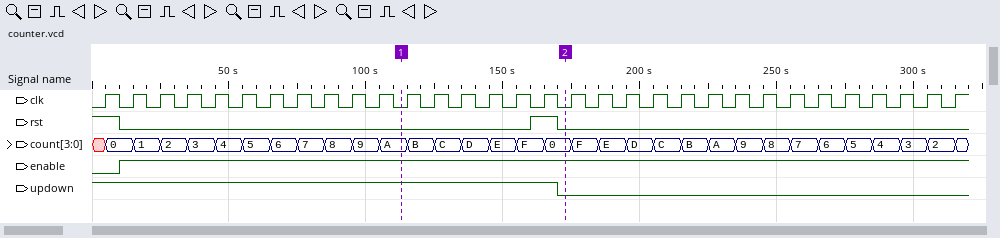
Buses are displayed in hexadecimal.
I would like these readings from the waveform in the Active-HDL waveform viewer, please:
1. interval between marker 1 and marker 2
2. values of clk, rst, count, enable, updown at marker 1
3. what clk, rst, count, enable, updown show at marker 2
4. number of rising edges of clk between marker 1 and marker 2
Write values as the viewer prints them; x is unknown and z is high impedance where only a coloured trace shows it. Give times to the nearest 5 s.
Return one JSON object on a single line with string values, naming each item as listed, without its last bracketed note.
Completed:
{"interval between marker 1 and marker 2": "60 s", "values of clk, rst, count, enable, updown at marker 1": "clk=0, rst=0, count=A, enable=1, updown=1", "what clk, rst, count, enable, updown show at marker 2": "clk=0, rst=0, count=0, enable=1, updown=0", "number of rising edges of clk between marker 1 and marker 2": "6"}
